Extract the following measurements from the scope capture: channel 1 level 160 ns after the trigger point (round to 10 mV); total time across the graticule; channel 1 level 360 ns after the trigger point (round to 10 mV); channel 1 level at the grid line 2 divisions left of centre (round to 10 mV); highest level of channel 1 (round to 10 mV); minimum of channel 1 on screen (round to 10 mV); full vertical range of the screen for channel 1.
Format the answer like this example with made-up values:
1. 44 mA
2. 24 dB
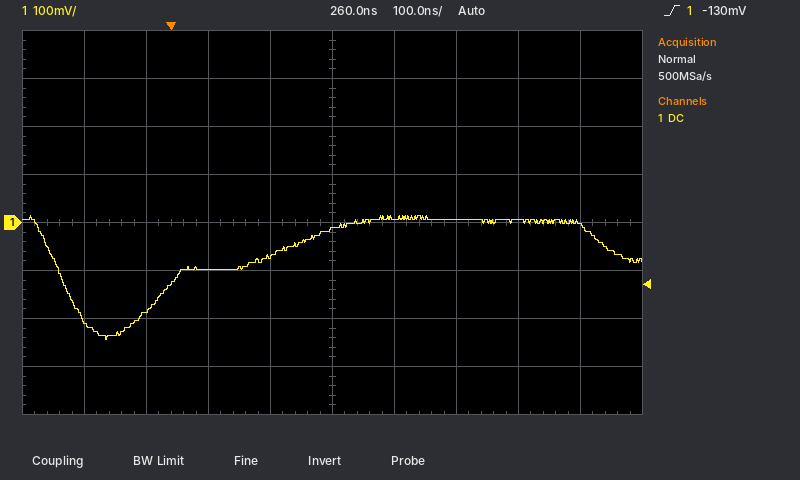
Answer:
1. -70 mV
2. 1 µs
3. 10 mV
4. -100 mV
5. 10 mV
6. -240 mV
7. 800 mV
